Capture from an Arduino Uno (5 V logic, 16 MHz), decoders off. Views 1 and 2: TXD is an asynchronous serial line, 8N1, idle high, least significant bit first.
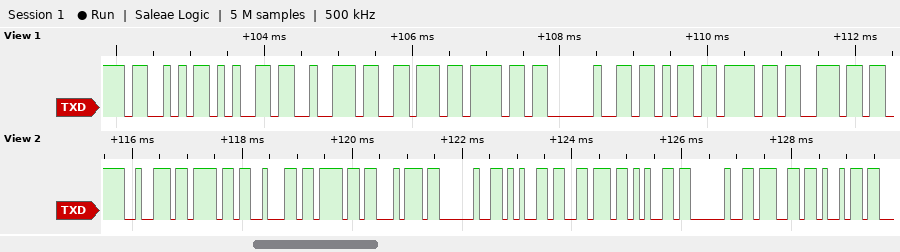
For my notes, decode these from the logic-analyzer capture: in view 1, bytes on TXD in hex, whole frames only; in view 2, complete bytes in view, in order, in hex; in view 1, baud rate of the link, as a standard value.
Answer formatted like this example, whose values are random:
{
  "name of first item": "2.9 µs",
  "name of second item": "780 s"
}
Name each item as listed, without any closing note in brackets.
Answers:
{
  "in view 1, bytes on TXD in hex, whole frames only": "0x53 0x65 0x72 0x76 0x6F 0x20 0x6B 0x6F 0x6E",
  "in view 2, complete bytes in view, in order, in hex": "72 6F 62 6F 74 20 65 76 65 20 67 69",
  "in view 1, baud rate of the link, as a standard value": "9600 baud"
}
